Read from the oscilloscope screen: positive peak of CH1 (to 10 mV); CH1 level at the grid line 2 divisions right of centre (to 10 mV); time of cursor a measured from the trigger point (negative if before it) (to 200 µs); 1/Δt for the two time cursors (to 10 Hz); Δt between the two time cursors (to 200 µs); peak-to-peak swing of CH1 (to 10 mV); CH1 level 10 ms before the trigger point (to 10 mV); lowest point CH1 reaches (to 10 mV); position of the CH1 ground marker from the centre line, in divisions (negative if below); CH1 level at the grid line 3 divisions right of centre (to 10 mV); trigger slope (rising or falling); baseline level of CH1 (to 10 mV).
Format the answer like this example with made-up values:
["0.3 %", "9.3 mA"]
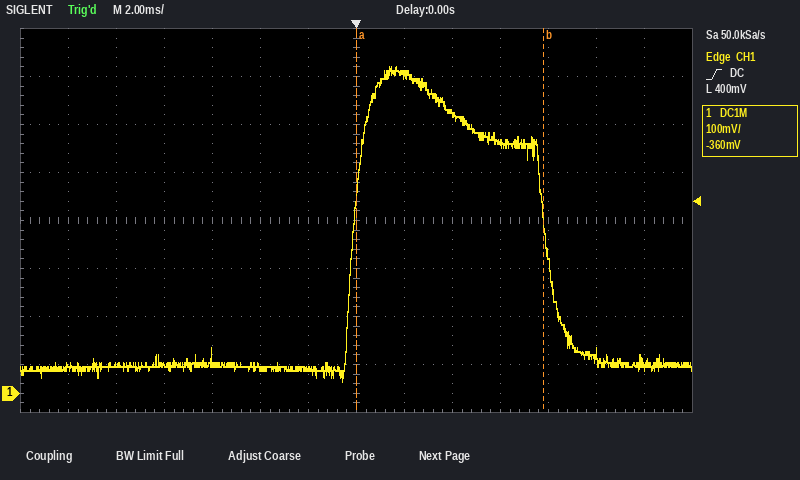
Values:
["680 mV", "580 mV", "0.0 ms", "130 Hz", "7.8 ms", "660 mV", "60 mV", "20 mV", "-3.6 div", "520 mV", "rising", "60 mV"]
